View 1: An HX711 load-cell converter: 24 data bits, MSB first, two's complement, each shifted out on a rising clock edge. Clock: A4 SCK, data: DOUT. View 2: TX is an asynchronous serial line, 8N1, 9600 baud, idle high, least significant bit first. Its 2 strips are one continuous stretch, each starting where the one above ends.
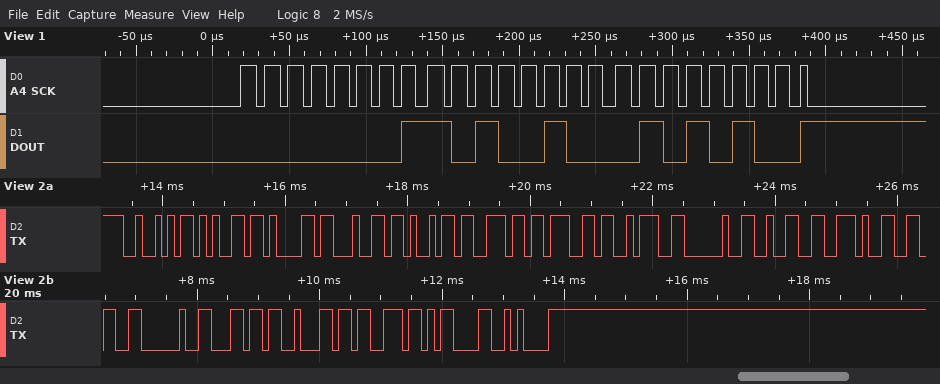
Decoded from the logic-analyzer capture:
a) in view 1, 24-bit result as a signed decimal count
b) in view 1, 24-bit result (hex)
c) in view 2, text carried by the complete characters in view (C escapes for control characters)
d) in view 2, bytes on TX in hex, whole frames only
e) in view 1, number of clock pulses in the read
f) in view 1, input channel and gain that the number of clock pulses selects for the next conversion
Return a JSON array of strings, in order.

["107604", "0x01A454", "\"Reading: 2.6 lbs\\r\\n\"", "0x52 0x65 0x61 0x64 0x69 0x6E 0x67 0x3A 0x20 0x32 0x2E 0x36 0x20 0x6C 0x62 0x73 0x0D 0x0A", "25", "channel A, gain 128"]
